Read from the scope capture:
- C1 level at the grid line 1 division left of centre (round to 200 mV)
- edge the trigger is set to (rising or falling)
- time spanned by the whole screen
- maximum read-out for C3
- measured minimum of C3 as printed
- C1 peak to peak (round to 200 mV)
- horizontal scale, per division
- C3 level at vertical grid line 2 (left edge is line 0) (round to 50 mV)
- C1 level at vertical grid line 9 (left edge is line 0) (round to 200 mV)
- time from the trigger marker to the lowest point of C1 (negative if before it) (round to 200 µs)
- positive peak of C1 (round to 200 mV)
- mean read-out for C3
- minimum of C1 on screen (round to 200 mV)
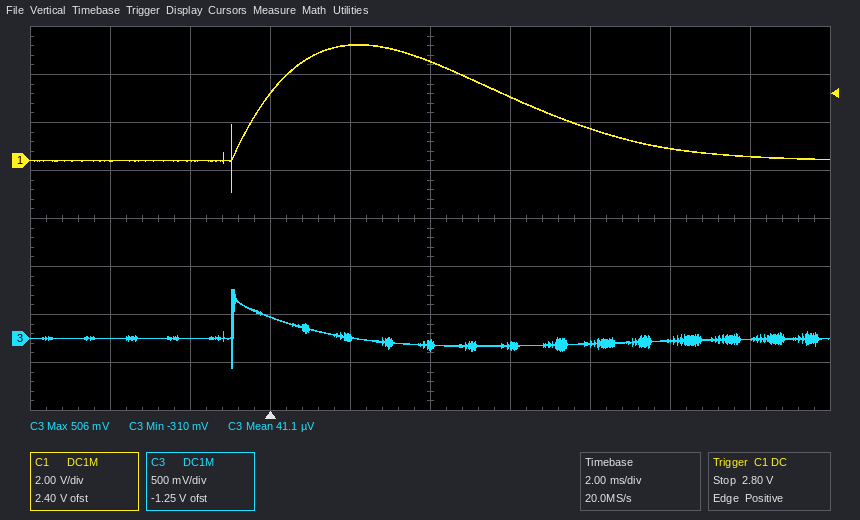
4.8 V
rising
20 ms
506 mV
-310 mV
6.2 V
2 ms
0 mV
200 mV
-1.0 ms
4.8 V
41.1 µV
-1.4 V
